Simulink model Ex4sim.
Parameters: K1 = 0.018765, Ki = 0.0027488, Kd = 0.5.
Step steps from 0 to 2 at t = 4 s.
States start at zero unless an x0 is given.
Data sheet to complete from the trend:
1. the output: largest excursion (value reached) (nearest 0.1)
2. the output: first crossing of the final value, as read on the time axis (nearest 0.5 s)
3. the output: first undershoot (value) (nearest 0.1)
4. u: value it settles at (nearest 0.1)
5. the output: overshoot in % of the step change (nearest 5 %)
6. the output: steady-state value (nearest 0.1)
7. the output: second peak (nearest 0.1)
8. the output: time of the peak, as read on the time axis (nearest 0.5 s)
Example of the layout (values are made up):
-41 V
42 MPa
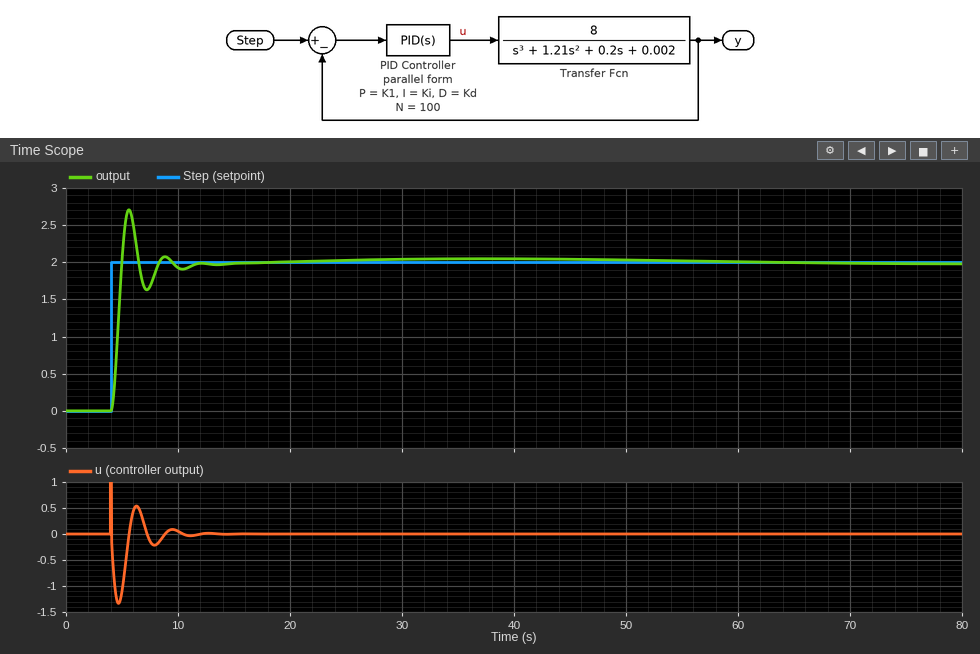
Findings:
2.7
5.0 s
1.6
0.0
35 %
2.0
2.1
5.5 s
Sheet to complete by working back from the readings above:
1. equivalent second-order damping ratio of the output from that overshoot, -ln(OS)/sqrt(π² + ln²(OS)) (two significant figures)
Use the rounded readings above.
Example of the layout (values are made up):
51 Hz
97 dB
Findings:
0.32
